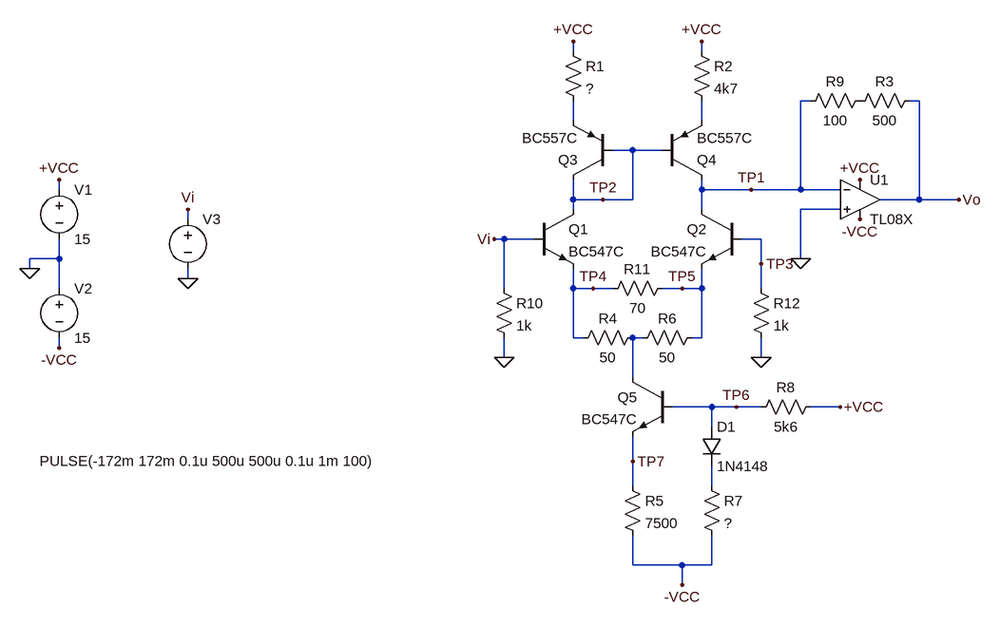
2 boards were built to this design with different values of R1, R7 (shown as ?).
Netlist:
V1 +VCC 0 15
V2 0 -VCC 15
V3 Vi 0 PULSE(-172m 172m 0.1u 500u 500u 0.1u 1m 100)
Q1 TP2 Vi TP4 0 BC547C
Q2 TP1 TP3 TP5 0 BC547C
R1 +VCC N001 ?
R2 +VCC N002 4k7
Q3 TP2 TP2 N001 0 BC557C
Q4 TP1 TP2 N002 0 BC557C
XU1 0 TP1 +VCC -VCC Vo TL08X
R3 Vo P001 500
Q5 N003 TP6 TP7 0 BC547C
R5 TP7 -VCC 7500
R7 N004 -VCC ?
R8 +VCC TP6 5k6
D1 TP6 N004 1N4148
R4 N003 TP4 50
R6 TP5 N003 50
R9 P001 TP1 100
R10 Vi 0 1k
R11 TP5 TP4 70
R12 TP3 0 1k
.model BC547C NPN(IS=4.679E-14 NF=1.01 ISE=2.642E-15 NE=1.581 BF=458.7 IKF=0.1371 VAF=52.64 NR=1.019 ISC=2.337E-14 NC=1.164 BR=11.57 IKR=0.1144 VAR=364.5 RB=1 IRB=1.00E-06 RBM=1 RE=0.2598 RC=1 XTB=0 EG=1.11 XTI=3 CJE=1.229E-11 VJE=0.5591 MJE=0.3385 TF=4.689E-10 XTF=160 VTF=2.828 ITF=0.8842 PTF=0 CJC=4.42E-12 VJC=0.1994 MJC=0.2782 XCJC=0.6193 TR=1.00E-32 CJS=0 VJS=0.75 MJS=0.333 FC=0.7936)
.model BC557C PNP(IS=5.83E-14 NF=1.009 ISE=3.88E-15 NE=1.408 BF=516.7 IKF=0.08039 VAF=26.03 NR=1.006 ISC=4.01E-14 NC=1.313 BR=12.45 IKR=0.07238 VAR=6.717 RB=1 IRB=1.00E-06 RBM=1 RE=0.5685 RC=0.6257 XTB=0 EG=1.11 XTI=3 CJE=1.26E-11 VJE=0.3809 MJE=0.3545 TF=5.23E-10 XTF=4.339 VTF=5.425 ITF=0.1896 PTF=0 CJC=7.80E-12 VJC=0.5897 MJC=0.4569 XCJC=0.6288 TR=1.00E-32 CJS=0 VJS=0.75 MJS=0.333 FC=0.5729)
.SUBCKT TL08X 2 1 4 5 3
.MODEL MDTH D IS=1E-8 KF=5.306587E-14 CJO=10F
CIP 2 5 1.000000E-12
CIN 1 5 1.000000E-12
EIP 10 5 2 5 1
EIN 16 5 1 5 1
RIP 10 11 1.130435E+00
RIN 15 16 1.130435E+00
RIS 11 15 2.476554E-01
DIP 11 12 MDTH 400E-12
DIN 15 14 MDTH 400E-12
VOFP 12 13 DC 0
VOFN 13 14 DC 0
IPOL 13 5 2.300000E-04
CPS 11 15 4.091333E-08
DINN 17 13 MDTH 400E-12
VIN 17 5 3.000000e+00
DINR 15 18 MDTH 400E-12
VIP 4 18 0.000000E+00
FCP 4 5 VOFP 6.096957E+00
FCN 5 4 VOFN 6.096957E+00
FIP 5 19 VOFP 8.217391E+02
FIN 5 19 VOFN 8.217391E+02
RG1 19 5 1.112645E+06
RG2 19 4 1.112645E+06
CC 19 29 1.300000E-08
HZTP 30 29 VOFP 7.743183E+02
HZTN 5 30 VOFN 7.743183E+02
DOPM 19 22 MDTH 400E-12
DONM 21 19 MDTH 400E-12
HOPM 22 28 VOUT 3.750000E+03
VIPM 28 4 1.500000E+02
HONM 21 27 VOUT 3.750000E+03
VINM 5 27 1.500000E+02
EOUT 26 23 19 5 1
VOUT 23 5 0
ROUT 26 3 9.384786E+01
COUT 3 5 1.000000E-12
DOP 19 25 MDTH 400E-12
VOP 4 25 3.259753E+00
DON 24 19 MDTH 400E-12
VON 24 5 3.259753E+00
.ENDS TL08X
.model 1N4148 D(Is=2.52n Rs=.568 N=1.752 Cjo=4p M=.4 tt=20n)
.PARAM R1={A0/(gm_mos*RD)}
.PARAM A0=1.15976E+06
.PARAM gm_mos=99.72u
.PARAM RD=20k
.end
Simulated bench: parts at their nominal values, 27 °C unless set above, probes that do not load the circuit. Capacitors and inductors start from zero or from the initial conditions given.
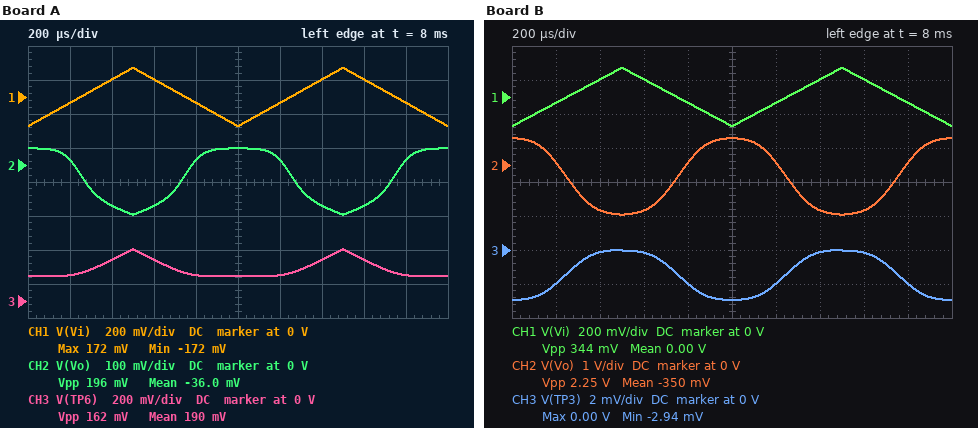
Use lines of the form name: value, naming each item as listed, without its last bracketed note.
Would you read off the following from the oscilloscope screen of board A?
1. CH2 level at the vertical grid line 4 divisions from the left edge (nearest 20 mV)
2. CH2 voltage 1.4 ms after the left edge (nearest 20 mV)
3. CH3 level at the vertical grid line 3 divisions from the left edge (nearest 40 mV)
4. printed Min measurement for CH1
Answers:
CH2 level at the vertical grid line 4 divisions from the left edge: 20 mV
CH2 voltage 1.4 ms after the left edge: -120 mV
CH3 level at the vertical grid line 3 divisions from the left edge: 240 mV
printed Min measurement for CH1: -172 mV
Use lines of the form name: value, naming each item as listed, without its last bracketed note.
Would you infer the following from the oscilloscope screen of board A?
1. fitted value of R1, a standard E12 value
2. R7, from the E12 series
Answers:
fitted value of R1, a standard E12 value: 8.2 kΩ
R7, from the E12 series: 18 kΩ
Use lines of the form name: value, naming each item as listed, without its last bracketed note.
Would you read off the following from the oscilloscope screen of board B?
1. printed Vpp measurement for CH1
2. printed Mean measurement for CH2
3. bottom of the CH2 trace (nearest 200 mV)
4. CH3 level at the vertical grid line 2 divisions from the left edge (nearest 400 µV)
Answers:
printed Vpp measurement for CH1: 344 mV
printed Mean measurement for CH2: -350 mV
bottom of the CH2 trace: -1.4 V
CH3 level at the vertical grid line 2 divisions from the left edge: 0 V
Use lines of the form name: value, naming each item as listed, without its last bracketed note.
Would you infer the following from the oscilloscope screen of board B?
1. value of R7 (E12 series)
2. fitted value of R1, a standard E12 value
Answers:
value of R7: 6.8 kΩ
fitted value of R1, a standard E12 value: 8.2 kΩ
